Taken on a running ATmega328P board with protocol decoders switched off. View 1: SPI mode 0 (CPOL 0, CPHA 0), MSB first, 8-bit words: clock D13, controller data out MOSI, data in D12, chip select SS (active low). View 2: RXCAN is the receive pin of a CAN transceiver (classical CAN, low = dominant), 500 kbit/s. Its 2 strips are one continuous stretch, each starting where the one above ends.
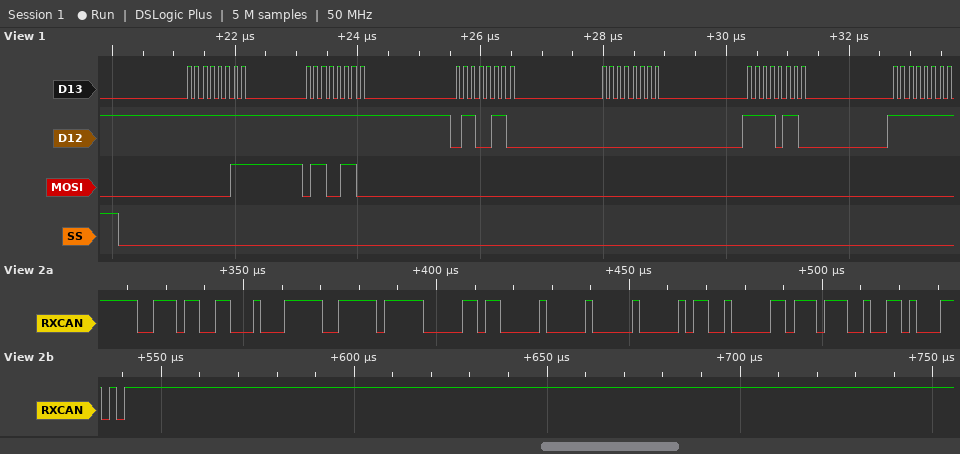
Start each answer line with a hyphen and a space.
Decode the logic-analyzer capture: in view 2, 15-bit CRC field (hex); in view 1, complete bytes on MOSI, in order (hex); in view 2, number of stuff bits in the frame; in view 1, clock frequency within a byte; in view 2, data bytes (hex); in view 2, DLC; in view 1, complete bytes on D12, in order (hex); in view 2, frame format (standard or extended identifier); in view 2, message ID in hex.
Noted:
- 0x1346
- 03 66 00 00 00 00
- 9
- 8 MHz
- FB FF 0B 00 00 06 41 77
- 8
- FF FF 66 00 F6 FF
- standard
- 0x3B3
